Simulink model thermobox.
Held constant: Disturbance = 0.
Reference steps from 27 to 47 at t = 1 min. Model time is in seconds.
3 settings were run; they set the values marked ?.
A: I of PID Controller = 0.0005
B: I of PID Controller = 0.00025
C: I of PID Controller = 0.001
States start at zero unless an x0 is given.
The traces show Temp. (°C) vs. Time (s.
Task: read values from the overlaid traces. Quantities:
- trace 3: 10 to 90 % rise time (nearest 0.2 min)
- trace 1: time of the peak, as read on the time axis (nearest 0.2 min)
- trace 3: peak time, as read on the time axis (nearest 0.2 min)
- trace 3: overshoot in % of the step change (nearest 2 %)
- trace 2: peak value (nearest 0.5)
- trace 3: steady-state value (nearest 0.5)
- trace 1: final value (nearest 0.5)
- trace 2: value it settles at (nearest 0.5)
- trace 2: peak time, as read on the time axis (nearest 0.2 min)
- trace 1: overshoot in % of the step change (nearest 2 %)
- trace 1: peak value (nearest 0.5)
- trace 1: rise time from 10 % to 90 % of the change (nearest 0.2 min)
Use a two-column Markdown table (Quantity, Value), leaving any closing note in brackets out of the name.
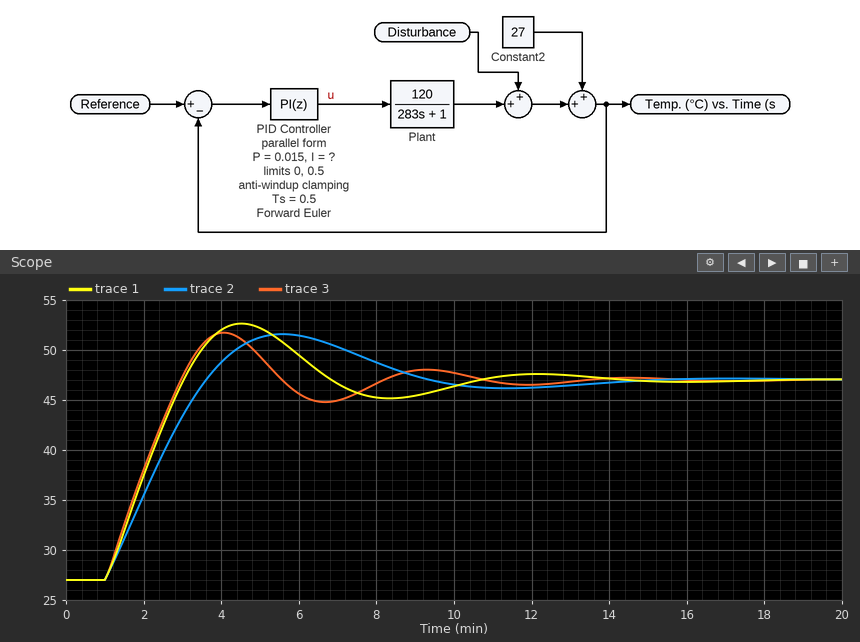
| Quantity | Value |
|---|---|
| trace 3: 10 to 90 % rise time | 1.6 min |
| trace 1: time of the peak, as read on the time axis | 4.6 min |
| trace 3: peak time, as read on the time axis | 4.0 min |
| trace 3: overshoot in % of the step change | 24 % |
| trace 2: peak value | 51.5 |
| trace 3: steady-state value | 47.0 |
| trace 1: final value | 47.0 |
| trace 2: value it settles at | 47.0 |
| trace 2: peak time, as read on the time axis | 5.6 min |
| trace 1: overshoot in % of the step change | 28 % |
| trace 1: peak value | 52.5 |
| trace 1: rise time from 10 % to 90 % of the change | 1.6 min |
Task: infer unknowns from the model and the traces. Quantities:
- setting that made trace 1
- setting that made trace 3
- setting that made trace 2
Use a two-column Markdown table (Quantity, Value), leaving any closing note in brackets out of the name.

| Quantity | Value |
|---|---|
| setting that made trace 1 | A |
| setting that made trace 3 | C |
| setting that made trace 2 | B |
